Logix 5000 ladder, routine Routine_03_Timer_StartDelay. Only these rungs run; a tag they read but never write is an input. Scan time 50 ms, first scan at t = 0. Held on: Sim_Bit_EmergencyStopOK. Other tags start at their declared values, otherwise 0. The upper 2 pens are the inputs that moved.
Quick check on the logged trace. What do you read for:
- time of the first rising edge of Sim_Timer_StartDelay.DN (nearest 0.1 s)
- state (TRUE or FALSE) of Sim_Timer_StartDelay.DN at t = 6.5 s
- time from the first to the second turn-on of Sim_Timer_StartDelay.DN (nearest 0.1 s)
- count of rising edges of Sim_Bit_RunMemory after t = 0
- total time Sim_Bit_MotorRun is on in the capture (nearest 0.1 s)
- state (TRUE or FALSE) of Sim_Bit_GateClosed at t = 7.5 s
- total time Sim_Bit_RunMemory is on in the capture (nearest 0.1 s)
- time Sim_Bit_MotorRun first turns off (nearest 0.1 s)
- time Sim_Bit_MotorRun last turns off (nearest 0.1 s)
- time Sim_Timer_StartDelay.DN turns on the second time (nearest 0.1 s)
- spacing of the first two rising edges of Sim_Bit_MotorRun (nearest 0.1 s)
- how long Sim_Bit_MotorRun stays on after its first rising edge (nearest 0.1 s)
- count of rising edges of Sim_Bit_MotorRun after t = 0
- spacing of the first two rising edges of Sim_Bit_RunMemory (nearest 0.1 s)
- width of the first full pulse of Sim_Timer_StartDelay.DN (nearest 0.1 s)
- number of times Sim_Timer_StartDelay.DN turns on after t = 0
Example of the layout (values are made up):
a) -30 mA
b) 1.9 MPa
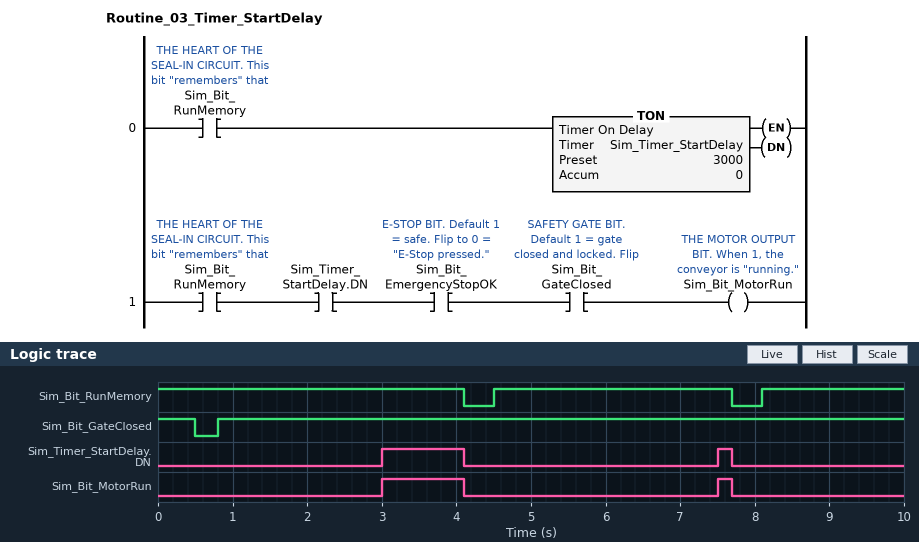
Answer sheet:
a) 3.0 s
b) FALSE
c) 4.5 s
d) 2
e) 1.3 s
f) TRUE
g) 9.2 s
h) 4.1 s
i) 7.7 s
j) 7.5 s
k) 4.5 s
l) 1.1 s
m) 2
n) 3.6 s
o) 1.1 s
p) 2
